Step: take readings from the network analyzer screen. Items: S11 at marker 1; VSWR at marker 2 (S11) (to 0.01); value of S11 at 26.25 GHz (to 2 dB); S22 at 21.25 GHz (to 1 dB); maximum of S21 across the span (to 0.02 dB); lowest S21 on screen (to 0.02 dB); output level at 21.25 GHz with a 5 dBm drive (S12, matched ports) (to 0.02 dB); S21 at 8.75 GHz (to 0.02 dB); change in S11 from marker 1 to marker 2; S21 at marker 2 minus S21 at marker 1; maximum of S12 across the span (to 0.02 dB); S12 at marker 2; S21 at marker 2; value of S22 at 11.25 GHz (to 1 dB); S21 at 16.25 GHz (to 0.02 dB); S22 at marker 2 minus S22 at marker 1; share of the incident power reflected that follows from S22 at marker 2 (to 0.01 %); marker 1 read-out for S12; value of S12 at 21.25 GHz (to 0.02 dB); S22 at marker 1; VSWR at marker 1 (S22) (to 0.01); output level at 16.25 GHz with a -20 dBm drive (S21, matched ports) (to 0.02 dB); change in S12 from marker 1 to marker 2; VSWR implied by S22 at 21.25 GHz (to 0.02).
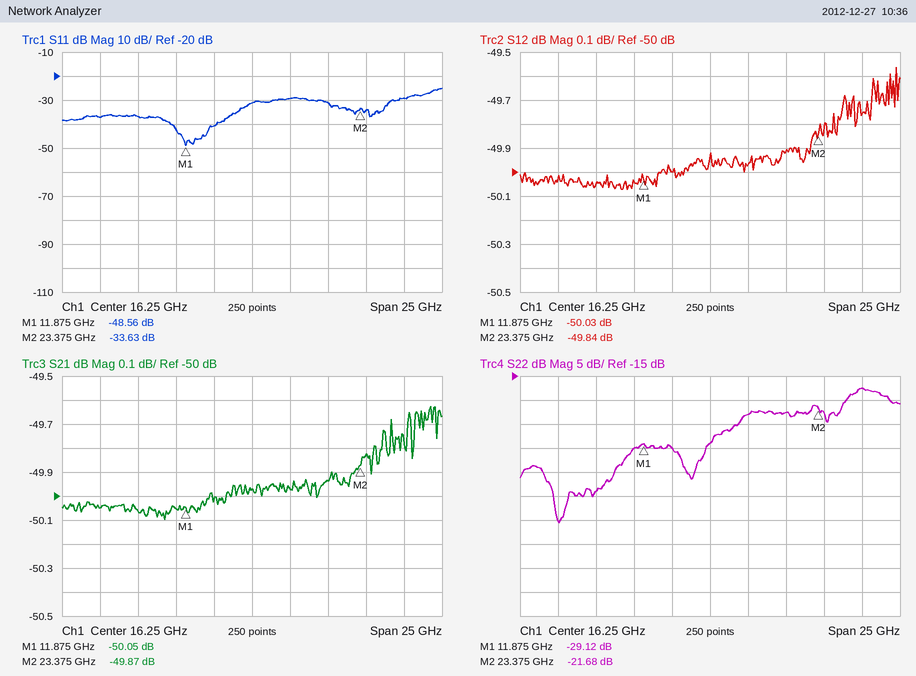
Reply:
-48.56 dB
1.04
-30 dB
-23 dB
-49.62 dB
-50.10 dB
-44.92 dBm
-50.06 dB
14.93 dB
0.18 dB
-49.56 dB
-49.84 dB
-49.87 dB
-30 dB
-49.98 dB
7.44 dB
0.68 %
-50.03 dB
-49.92 dB
-29.12 dB
1.07
-69.98 dBm
0.19 dB
1.16
